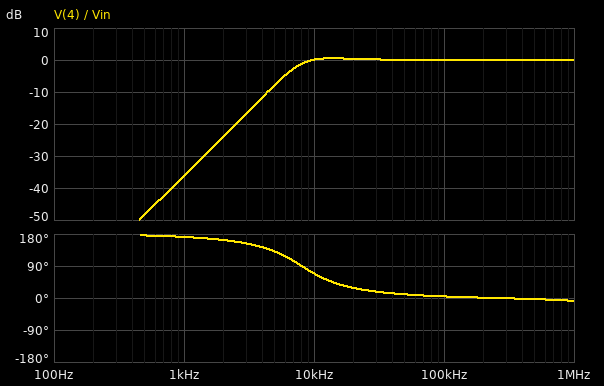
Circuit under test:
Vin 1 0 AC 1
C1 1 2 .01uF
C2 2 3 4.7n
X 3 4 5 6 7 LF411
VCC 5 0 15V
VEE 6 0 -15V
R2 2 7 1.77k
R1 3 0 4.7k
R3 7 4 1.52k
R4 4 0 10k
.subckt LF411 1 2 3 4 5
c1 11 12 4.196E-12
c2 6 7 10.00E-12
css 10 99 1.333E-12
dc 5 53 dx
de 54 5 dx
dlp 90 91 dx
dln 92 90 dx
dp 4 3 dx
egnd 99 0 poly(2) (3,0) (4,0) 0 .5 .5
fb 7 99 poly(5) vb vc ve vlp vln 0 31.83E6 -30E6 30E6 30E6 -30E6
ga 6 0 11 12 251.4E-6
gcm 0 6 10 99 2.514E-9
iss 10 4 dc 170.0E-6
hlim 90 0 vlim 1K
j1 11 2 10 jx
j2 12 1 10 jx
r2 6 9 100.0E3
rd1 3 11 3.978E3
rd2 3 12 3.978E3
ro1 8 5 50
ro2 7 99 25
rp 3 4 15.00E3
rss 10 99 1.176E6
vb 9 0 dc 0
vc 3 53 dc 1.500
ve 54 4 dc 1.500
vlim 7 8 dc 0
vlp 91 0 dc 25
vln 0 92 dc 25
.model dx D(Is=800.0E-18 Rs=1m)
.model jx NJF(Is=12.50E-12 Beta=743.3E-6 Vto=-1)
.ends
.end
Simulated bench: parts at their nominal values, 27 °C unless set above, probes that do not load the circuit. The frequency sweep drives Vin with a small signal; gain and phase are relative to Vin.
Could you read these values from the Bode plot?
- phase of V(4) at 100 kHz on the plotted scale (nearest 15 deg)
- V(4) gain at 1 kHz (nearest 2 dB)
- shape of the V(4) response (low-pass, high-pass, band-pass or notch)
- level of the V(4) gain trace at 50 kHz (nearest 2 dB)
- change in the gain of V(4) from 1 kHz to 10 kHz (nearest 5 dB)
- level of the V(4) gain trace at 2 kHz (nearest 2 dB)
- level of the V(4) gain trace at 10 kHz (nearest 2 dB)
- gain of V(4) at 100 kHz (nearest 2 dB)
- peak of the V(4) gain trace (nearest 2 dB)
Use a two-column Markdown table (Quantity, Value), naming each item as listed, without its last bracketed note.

| Quantity | Value |
|---|---|
| phase of V(4) at 100 kHz on the plotted scale | 0 deg |
| V(4) gain at 1 kHz | -36 dB |
| shape of the V(4) response | high-pass |
| level of the V(4) gain trace at 50 kHz | 0 dB |
| change in the gain of V(4) from 1 kHz to 10 kHz | 35 dB |
| level of the V(4) gain trace at 2 kHz | -24 dB |
| level of the V(4) gain trace at 10 kHz | 0 dB |
| gain of V(4) at 100 kHz | 0 dB |
| peak of the V(4) gain trace | 0 dB |
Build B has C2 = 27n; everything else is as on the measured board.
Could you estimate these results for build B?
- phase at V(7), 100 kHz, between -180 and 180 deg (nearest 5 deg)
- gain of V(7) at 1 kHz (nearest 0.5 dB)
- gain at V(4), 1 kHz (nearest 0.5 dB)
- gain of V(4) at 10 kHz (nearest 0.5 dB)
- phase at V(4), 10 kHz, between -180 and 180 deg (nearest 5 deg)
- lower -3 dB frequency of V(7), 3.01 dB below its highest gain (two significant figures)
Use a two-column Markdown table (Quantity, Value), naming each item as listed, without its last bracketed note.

| Quantity | Value |
|---|---|
| phase at V(7), 100 kHz, between -180 and 180 deg | 0 deg |
| gain of V(7) at 1 kHz | -19.5 dB |
| gain at V(4), 1 kHz | -20.5 dB |
| gain of V(4) at 10 kHz | 0.5 dB |
| phase at V(4), 10 kHz, between -180 and 180 deg | 20 deg |
| lower -3 dB frequency of V(7), 3.01 dB below its highest gain | 3.0 kHz |
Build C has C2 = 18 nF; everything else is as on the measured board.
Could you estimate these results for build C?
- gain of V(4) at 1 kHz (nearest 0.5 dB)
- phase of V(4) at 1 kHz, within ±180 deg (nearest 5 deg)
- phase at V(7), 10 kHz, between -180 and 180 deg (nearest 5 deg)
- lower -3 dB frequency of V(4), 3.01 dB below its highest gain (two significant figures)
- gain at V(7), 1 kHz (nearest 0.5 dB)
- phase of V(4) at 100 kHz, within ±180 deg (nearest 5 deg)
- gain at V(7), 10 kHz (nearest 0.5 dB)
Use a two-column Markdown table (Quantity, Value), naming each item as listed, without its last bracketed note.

| Quantity | Value |
|---|---|
| gain of V(4) at 1 kHz | -24.5 dB |
| phase of V(4) at 1 kHz, within ±180 deg | 165 deg |
| phase at V(7), 10 kHz, between -180 and 180 deg | 25 deg |
| lower -3 dB frequency of V(4), 3.01 dB below its highest gain | 3.7 kHz |
| gain at V(7), 1 kHz | -23.0 dB |
| phase of V(4) at 100 kHz, within ±180 deg | 0 deg |
| gain at V(7), 10 kHz | 2.0 dB |
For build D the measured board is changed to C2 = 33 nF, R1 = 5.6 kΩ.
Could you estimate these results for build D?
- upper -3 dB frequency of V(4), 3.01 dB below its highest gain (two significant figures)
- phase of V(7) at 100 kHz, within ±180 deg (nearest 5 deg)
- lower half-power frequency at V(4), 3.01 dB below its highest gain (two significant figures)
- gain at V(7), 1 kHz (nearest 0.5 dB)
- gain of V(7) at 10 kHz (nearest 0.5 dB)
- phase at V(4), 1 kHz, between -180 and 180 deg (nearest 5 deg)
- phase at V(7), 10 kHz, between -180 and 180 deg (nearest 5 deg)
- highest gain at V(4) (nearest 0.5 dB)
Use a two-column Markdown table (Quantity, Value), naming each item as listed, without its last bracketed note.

| Quantity | Value |
|---|---|
| upper -3 dB frequency of V(4), 3.01 dB below its highest gain | 6.6 MHz |
| phase of V(7) at 100 kHz, within ±180 deg | 0 deg |
| lower half-power frequency at V(4), 3.01 dB below its highest gain | 2.3 kHz |
| gain at V(7), 1 kHz | -16.0 dB |
| gain of V(7) at 10 kHz | 1.5 dB |
| phase at V(4), 1 kHz, between -180 and 180 deg | 160 deg |
| phase at V(7), 10 kHz, between -180 and 180 deg | 15 deg |
| highest gain at V(4) | 2.5 dB |
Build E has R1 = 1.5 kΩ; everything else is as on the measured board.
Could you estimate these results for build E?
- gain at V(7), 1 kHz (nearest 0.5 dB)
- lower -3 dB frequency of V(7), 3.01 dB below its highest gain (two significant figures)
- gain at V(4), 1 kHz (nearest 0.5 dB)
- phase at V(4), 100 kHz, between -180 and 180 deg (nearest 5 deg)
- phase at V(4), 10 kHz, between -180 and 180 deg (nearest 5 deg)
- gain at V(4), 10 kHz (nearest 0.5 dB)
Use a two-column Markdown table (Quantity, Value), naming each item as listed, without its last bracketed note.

| Quantity | Value |
|---|---|
| gain at V(7), 1 kHz | -45.0 dB |
| lower -3 dB frequency of V(7), 3.01 dB below its highest gain | 55 kHz |
| gain at V(4), 1 kHz | -46.0 dB |
| phase at V(4), 100 kHz, between -180 and 180 deg | 15 deg |
| phase at V(4), 10 kHz, between -180 and 180 deg | 110 deg |
| gain at V(4), 10 kHz | -10.5 dB |
